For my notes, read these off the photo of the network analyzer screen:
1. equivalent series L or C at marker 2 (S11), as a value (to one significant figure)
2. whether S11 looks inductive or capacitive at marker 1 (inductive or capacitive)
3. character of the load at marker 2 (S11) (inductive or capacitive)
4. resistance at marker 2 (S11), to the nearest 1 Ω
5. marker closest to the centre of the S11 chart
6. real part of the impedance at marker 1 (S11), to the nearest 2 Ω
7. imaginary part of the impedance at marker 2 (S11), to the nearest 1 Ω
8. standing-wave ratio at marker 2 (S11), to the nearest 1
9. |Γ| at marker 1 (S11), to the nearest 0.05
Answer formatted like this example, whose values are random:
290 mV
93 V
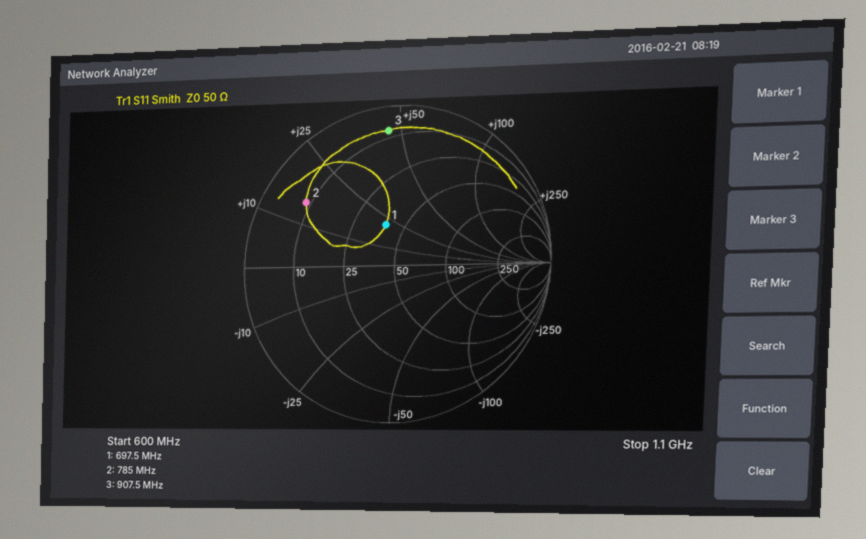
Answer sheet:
3 nH
inductive
inductive
9 Ω
marker 1
38 Ω
+15 Ω
6
0.25
